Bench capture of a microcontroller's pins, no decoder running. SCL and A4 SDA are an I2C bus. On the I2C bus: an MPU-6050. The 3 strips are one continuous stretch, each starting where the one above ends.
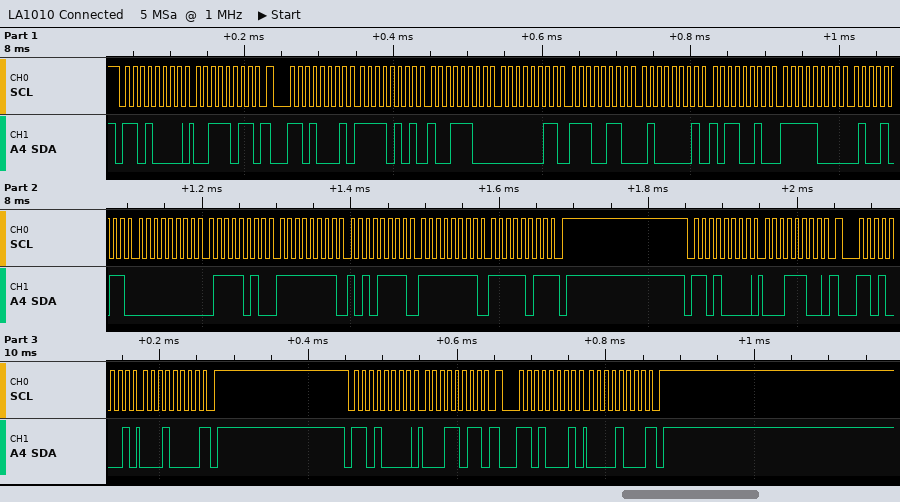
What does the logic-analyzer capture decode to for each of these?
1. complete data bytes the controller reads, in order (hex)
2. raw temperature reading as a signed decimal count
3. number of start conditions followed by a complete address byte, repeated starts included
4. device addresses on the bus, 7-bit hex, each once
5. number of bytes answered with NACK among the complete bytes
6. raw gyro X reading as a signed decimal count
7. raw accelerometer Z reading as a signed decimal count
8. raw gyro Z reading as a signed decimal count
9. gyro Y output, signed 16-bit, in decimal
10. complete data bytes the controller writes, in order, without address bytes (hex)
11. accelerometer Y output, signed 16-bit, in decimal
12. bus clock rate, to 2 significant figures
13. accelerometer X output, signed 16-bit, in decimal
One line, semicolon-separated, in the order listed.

F5 9C 03 E6 41 B2 F8 4B 00 7A FF AF FF FB 10 08; -1973; 6; 0x68; 3; 122; 16818; -5; -81; 3B 1C 1B; 998; 100 kHz; -2660
